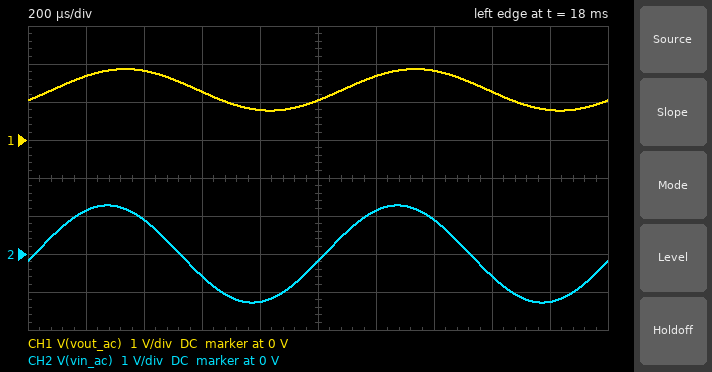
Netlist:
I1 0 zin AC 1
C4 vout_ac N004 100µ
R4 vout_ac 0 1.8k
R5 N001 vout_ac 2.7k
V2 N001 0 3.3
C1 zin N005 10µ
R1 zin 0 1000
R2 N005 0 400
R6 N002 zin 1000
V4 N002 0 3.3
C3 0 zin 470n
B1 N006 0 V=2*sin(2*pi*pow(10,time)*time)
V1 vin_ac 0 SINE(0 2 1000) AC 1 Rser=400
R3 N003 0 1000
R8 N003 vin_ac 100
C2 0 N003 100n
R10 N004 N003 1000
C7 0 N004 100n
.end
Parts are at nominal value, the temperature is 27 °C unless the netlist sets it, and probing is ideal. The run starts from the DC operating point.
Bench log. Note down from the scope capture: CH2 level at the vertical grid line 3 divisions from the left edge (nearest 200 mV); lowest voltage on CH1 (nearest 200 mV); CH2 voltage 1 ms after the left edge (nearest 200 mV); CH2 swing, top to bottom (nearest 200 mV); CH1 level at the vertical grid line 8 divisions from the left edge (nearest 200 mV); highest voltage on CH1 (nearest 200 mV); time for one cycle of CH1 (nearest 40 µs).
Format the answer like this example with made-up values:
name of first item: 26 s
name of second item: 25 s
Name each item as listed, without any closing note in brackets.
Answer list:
CH2 level at the vertical grid line 3 divisions from the left edge: -600 mV
lowest voltage on CH1: 800 mV
CH2 voltage 1 ms after the left edge: -200 mV
CH2 swing, top to bottom: 2.6 V
CH1 level at the vertical grid line 8 divisions from the left edge: 1.2 V
highest voltage on CH1: 1.8 V
time for one cycle of CH1: 1.00 ms
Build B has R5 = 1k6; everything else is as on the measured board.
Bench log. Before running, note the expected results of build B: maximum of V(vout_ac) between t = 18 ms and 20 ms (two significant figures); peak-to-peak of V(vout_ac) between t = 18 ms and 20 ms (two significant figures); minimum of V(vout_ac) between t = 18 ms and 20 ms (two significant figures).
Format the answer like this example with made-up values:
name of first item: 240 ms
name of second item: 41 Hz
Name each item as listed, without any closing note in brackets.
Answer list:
maximum of V(vout_ac) between t = 18 ms and 20 ms: 2.2 V
peak-to-peak of V(vout_ac) between t = 18 ms and 20 ms: 960 mV
minimum of V(vout_ac) between t = 18 ms and 20 ms: 1.3 V
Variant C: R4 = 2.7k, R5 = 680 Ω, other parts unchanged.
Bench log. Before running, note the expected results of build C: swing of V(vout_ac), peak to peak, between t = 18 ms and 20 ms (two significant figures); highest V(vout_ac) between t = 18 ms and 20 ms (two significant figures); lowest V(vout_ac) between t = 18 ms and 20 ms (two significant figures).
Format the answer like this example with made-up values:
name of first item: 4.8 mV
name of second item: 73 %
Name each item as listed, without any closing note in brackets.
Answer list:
swing of V(vout_ac), peak to peak, between t = 18 ms and 20 ms: 740 mV
highest V(vout_ac) between t = 18 ms and 20 ms: 3.0 V
lowest V(vout_ac) between t = 18 ms and 20 ms: 2.3 V
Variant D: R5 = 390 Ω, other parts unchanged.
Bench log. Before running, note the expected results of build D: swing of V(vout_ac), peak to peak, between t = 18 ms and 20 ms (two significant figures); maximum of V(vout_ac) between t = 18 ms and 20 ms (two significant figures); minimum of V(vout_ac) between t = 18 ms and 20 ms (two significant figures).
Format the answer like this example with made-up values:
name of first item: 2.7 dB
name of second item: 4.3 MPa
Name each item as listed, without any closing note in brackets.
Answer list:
swing of V(vout_ac), peak to peak, between t = 18 ms and 20 ms: 500 mV
maximum of V(vout_ac) between t = 18 ms and 20 ms: 3.0 V
minimum of V(vout_ac) between t = 18 ms and 20 ms: 2.5 V
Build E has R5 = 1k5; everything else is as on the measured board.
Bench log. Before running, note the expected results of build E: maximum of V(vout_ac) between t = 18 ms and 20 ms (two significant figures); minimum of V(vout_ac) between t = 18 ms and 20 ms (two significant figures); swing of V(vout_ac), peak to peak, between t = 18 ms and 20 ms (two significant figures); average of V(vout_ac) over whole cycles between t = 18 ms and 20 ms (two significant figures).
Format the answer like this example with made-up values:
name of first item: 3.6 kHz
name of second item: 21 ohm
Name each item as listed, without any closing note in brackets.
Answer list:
maximum of V(vout_ac) between t = 18 ms and 20 ms: 2.3 V
minimum of V(vout_ac) between t = 18 ms and 20 ms: 1.3 V
swing of V(vout_ac), peak to peak, between t = 18 ms and 20 ms: 950 mV
average of V(vout_ac) over whole cycles between t = 18 ms and 20 ms: 1.8 V
